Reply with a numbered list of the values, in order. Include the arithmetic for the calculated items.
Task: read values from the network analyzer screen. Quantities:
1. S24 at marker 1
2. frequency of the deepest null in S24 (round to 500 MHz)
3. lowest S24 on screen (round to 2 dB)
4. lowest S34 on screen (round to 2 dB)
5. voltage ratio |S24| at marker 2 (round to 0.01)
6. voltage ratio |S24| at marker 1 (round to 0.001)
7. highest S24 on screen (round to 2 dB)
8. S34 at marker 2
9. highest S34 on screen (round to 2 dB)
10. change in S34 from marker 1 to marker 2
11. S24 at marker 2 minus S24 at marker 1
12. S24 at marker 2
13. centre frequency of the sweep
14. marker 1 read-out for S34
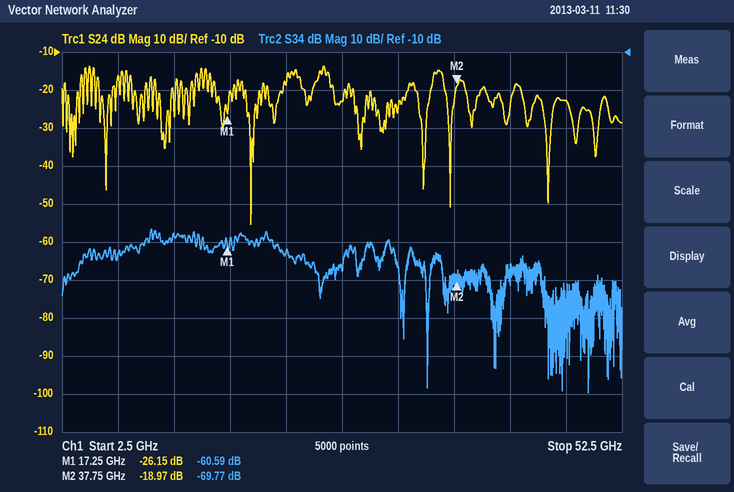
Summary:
1. -26.15 dB
2. 19.5 GHz
3. -56 dB
4. -100 dB
5. 10^(-18.97/20) ≈ 0.11
6. 10^(-26.15/20) ≈ 0.049
7. -14 dB
8. -69.77 dB
9. -56 dB
10. -69.77 − (-60.59) = -9.18 dB
11. -18.97 − (-26.15) = 7.18 dB
12. -18.97 dB
13. 27.5 GHz
14. -60.59 dB
